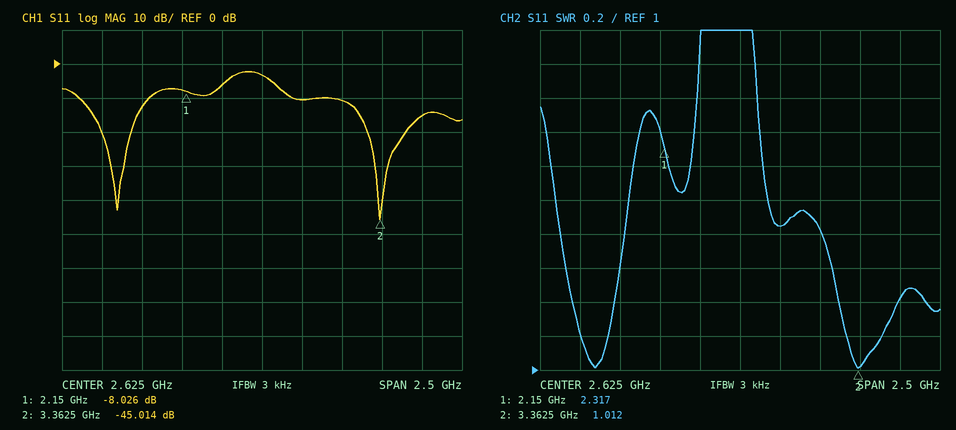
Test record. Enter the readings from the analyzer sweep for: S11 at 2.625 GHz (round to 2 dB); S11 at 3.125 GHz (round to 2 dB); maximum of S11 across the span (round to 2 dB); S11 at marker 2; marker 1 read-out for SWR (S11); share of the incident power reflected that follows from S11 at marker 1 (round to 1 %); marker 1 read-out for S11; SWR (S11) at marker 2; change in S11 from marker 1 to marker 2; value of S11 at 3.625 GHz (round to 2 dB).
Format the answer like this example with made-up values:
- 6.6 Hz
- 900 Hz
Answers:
- -4 dB
- -10 dB
- -2 dB
- -45.014 dB
- 2.317
- 16 %
- -8.026 dB
- 1.012
- -36.988 dB
- -16 dB
